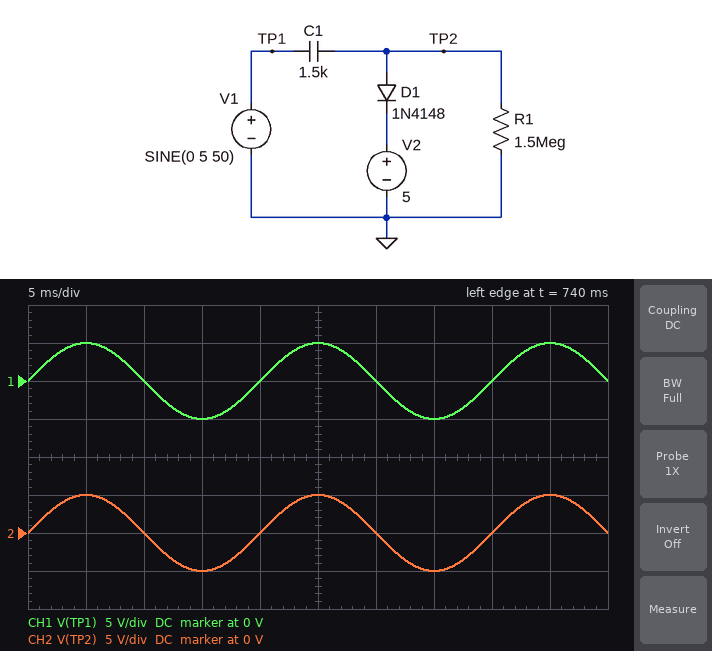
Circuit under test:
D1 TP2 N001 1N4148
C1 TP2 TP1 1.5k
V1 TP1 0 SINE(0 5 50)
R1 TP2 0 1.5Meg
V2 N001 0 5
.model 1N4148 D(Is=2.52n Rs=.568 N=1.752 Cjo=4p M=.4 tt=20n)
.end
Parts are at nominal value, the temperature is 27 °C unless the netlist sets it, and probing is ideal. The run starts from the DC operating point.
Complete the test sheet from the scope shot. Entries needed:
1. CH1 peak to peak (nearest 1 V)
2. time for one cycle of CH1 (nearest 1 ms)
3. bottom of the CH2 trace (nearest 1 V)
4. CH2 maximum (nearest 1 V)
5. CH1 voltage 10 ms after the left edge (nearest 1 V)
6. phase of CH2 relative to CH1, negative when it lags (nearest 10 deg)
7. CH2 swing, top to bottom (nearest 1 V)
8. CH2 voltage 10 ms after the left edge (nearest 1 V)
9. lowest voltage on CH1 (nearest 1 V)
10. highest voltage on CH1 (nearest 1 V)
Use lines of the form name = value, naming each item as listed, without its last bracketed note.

CH1 peak to peak = 10 V
time for one cycle of CH1 = 20 ms
bottom of the CH2 trace = -5 V
CH2 maximum = 5 V
CH1 voltage 10 ms after the left edge = 0 V
phase of CH2 relative to CH1, negative when it lags = 0 deg
CH2 swing, top to bottom = 10 V
CH2 voltage 10 ms after the left edge = 0 V
lowest voltage on CH1 = -5 V
highest voltage on CH1 = 5 V
